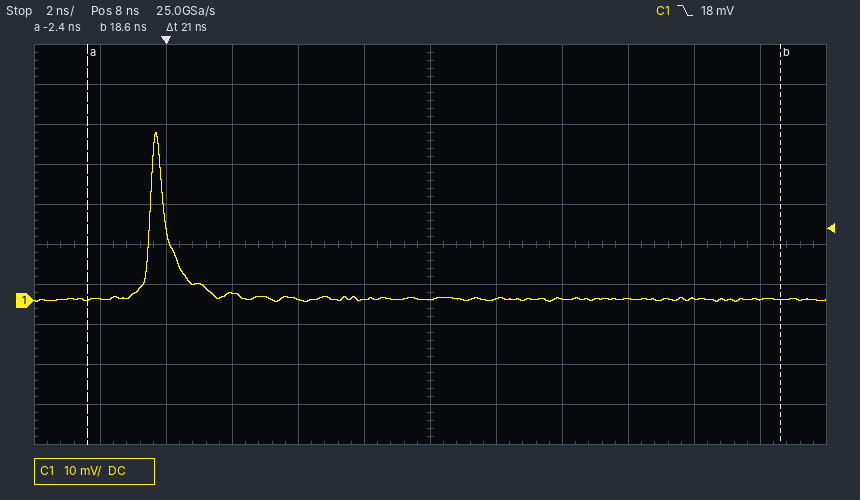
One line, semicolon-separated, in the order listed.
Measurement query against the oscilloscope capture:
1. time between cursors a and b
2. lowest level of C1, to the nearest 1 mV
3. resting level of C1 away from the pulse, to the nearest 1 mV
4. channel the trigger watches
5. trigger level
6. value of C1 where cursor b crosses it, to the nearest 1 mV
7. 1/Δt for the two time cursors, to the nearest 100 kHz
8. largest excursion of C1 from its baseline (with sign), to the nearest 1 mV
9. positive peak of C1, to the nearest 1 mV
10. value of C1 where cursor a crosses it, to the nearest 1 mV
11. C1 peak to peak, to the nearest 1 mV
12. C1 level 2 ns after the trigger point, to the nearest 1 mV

21 ns; 0 mV; 0 mV; C1; 18 mV; 0 mV; 47.6 MHz; +42 mV; 42 mV; 0 mV; 42 mV; 2 mV
